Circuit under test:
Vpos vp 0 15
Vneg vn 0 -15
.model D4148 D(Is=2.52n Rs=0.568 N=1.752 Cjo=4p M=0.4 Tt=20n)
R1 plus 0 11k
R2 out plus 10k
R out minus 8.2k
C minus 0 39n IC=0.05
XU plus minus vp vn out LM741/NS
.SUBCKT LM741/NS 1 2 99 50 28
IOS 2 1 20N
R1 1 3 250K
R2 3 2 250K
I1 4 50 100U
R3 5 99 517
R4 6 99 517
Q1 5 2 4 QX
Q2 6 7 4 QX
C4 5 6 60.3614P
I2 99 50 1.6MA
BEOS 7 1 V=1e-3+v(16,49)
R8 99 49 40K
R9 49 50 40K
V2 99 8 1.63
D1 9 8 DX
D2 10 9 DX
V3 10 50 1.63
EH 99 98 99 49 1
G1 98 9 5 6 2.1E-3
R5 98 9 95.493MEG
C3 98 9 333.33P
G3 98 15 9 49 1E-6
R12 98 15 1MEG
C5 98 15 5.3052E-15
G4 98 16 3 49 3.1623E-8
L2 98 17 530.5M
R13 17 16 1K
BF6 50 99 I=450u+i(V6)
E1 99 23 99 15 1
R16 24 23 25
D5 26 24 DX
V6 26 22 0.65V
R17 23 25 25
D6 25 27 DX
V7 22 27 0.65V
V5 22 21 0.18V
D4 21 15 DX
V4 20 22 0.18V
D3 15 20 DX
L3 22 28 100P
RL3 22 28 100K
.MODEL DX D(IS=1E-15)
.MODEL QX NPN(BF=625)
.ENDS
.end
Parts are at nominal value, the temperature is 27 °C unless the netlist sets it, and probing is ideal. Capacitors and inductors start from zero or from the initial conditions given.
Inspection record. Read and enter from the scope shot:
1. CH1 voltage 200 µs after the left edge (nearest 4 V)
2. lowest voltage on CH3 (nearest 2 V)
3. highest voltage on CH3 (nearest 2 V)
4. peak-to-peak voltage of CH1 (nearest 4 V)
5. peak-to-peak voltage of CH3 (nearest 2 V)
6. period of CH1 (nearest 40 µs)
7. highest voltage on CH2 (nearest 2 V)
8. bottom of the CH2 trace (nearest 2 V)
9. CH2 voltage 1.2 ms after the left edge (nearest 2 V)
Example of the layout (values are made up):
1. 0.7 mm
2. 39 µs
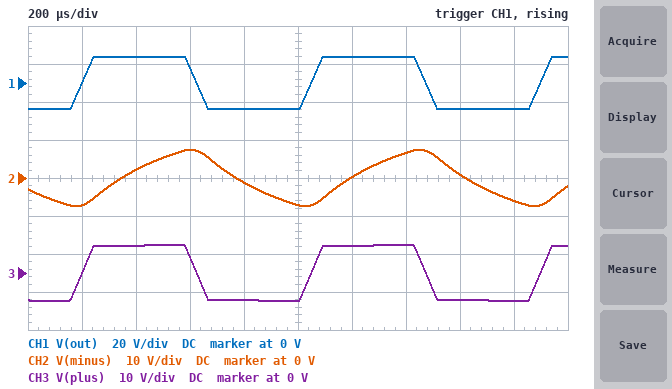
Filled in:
1. 0 V
2. -8 V
3. 8 V
4. 28 V
5. 14 V
6. 840 µs
7. 8 V
8. -8 V
9. 0 V
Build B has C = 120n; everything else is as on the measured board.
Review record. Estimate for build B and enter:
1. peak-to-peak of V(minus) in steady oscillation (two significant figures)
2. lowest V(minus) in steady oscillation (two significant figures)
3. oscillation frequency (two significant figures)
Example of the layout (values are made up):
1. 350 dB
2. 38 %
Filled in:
1. 15 V
2. -7.3 V
3. 420 Hz
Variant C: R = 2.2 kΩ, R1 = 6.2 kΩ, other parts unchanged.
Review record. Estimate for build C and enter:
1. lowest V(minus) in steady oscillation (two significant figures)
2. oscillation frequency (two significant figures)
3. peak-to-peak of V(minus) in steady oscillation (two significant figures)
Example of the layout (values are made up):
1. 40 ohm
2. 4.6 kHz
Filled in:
1. -6.4 V
2. 3.8 kHz
3. 13 V
